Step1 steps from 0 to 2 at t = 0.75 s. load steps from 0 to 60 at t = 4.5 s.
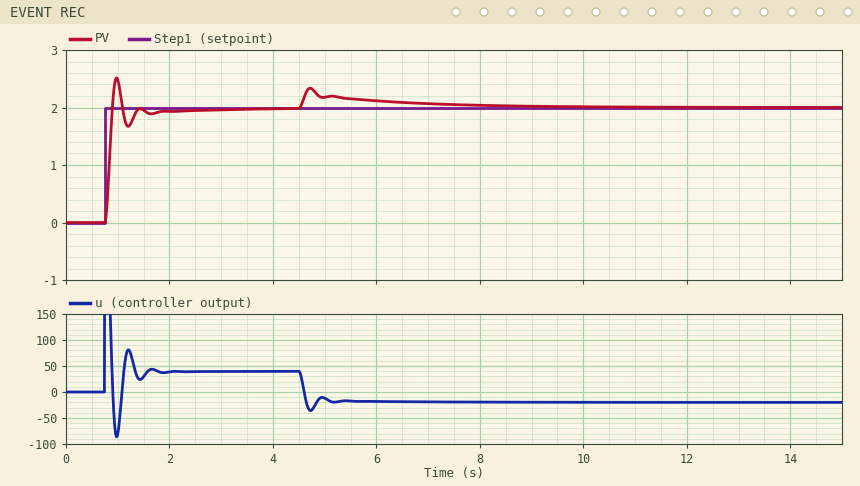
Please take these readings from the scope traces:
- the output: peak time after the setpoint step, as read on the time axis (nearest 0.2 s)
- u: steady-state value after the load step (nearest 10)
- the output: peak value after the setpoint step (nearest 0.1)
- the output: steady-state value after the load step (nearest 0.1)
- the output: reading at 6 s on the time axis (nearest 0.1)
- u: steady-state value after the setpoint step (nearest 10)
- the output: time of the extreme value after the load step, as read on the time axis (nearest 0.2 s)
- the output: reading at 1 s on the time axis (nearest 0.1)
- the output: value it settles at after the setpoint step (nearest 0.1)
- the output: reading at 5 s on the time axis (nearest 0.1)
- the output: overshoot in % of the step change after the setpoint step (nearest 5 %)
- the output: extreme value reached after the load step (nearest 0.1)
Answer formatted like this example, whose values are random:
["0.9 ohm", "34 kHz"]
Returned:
["1.0 s", "-20", "2.5", "2.0", "2.1", "40", "4.8 s", "2.5", "2.0", "2.2", "25 %", "2.3"]
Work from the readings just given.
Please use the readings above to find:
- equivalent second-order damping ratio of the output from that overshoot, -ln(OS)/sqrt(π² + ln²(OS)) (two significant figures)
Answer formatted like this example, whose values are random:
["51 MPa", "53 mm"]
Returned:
["0.40"]
